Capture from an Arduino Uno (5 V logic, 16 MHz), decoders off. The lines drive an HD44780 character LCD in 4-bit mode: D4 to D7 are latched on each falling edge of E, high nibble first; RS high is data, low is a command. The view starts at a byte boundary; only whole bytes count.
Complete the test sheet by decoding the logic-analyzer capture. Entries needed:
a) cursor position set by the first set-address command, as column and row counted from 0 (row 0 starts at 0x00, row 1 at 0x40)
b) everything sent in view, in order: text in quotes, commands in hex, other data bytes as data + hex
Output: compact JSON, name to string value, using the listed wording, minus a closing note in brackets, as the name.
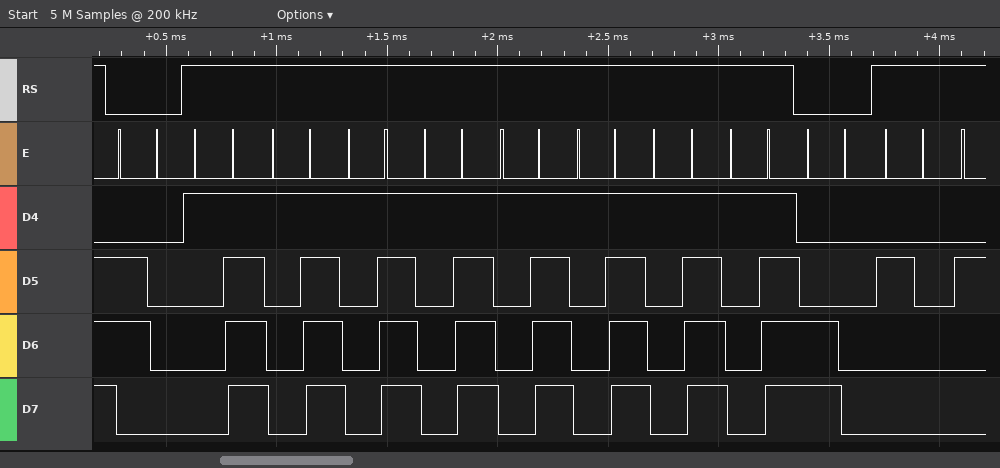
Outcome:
{"cursor position set by the first set-address command, as column and row counted from 0": "column 0, row 1", "everything sent in view, in order: text in quotes, commands in hex, other data bytes as data + hex": "0x60 data 1F 1F 1F 1F 1F 1F 1F 1F 0xC0 \" \""}
